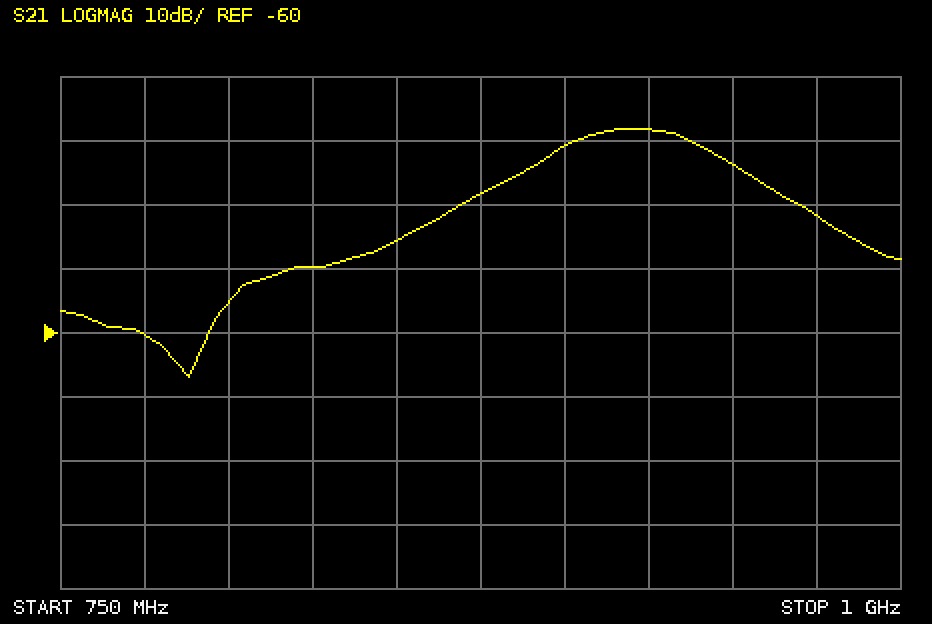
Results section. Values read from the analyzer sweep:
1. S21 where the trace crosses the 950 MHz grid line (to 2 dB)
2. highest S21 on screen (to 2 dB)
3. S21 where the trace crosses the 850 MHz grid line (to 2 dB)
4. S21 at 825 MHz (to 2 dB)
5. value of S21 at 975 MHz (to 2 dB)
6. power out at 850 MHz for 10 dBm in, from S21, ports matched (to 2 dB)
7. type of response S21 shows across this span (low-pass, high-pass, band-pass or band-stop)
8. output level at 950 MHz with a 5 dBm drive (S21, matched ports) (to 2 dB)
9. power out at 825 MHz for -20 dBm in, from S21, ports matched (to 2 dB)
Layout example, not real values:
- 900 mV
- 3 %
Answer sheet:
- -34 dB
- -28 dB
- -46 dB
- -50 dB
- -42 dB
- -36 dBm
- band-pass
- -28 dBm
- -70 dBm
